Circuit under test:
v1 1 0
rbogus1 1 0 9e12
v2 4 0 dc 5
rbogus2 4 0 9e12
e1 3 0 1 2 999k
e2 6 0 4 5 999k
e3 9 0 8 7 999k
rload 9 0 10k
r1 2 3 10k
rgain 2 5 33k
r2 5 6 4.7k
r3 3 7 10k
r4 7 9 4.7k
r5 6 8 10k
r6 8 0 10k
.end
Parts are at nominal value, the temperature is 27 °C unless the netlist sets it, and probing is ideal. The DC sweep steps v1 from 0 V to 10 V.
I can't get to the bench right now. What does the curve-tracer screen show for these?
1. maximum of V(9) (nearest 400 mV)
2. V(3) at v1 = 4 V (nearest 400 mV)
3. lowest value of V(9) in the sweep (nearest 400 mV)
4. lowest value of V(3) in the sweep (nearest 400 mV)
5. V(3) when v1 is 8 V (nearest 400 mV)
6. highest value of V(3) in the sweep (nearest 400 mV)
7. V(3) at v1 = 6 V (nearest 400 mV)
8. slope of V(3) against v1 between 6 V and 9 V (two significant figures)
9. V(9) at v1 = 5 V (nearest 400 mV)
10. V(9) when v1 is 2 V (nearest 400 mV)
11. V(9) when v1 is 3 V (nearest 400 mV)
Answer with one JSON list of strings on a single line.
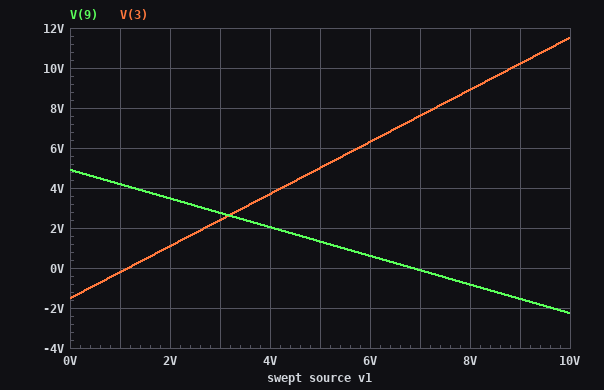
["4.8 V", "3.6 V", "-2.4 V", "-1.6 V", "8.8 V", "11.6 V", "6.4 V", "1.3 V/V", "1.2 V", "3.6 V", "2.8 V"]
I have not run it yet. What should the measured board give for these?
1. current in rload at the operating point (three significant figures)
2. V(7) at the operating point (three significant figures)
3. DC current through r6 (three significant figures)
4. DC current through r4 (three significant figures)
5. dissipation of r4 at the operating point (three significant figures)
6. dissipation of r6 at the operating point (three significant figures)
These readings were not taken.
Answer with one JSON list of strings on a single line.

["491 µA", "2.86 V", "286 µA", "437 µA", "898 µW", "816 µW"]
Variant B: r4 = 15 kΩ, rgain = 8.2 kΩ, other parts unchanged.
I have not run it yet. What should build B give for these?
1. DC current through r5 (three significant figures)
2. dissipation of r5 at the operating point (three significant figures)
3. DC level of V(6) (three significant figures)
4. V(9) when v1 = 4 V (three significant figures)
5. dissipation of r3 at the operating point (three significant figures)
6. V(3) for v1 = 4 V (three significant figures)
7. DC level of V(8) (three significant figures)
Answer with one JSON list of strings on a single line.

["393 µA", "1.55 mW", "7.87 V", "2.80 V", "10.1 mW", "2.78 V", "3.93 V"]
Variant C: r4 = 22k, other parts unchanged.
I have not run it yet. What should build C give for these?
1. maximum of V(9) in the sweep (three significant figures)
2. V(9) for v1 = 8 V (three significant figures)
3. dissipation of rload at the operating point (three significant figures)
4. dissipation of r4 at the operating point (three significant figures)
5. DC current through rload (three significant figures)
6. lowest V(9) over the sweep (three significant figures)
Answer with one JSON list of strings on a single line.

["12.5 V", "-12.3 V", "15.6 mW", "4.20 mW", "1.25 mA", "-18.5 V"]
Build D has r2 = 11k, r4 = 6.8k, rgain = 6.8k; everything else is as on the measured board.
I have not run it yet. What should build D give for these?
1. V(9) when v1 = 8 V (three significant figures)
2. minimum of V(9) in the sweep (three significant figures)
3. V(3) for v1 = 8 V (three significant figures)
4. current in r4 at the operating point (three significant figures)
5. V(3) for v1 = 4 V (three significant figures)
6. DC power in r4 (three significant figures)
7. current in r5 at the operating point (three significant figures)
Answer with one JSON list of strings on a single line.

["-8.32 V", "-14.4 V", "12.4 V", "1.39 mA", "2.53 V", "13.1 mW", "654 µA"]
